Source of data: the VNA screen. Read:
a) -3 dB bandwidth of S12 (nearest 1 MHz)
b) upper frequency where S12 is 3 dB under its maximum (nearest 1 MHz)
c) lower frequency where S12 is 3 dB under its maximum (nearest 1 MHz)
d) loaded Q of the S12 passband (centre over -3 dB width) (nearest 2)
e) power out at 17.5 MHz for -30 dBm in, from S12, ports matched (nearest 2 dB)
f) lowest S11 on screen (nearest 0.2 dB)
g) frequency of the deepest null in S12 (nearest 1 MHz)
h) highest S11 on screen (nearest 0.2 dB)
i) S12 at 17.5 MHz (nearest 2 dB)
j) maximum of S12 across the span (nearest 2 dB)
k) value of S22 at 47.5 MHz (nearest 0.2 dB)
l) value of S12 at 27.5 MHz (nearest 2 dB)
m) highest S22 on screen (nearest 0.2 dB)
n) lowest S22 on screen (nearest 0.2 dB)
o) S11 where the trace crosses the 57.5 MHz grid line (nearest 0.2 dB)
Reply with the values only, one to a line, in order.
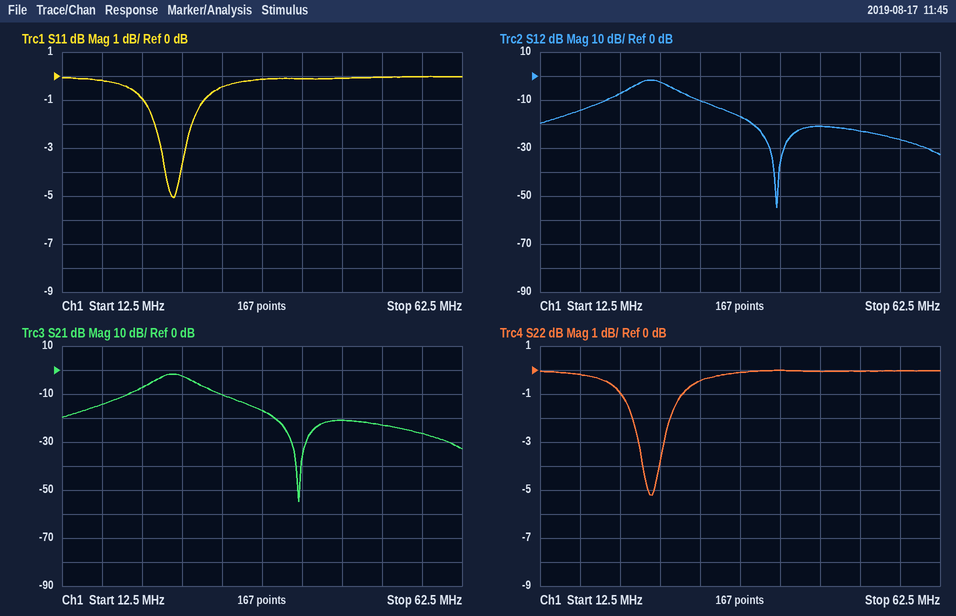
5 MHz
29 MHz
24 MHz
6
-44 dBm
-5.0 dB
42 MHz
0.0 dB
-14 dB
-2 dB
0.0 dB
-2 dB
0.0 dB
-5.2 dB
0.0 dB
